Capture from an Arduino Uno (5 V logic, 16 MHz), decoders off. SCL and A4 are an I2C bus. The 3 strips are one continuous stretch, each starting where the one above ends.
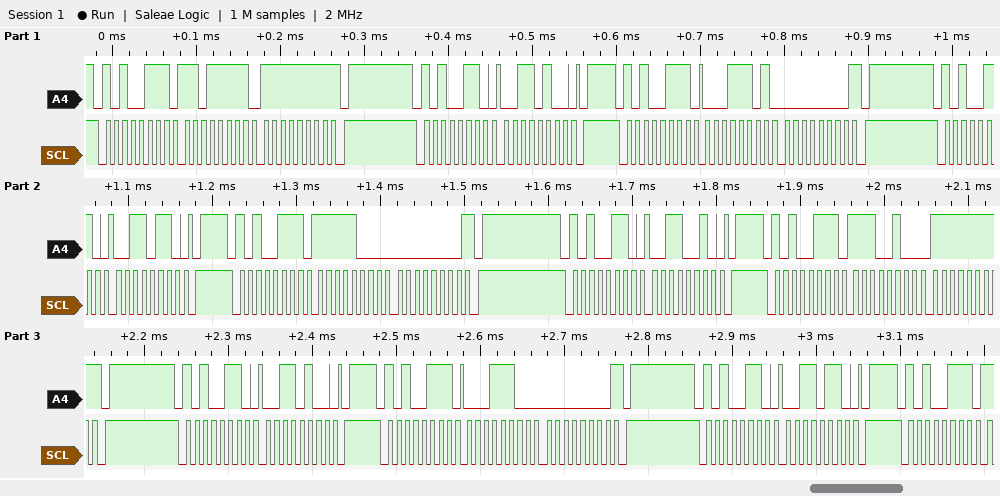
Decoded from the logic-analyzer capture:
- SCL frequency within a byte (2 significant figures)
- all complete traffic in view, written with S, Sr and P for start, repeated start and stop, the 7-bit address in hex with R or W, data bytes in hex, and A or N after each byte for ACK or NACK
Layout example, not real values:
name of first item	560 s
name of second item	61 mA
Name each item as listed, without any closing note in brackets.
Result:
SCL frequency within a byte	100 kHz
all complete traffic in view, written with S, Sr and P for start, repeated start and stop, the 7-bit address in hex with R or W, data bytes in hex, and A or N after each byte for ACK or NACK	S 53R A DF A FF N P S 53W A 34 A P S 53R A 1D A 00 N P S 53W A 36 A P S 53R A F8 A 00 N P S 53W A 32 A P S 53R A E4 A FF N P S 53W A 34 A P S 53R A 1C A 00 N P S 53W A 36 A P S 53R A
